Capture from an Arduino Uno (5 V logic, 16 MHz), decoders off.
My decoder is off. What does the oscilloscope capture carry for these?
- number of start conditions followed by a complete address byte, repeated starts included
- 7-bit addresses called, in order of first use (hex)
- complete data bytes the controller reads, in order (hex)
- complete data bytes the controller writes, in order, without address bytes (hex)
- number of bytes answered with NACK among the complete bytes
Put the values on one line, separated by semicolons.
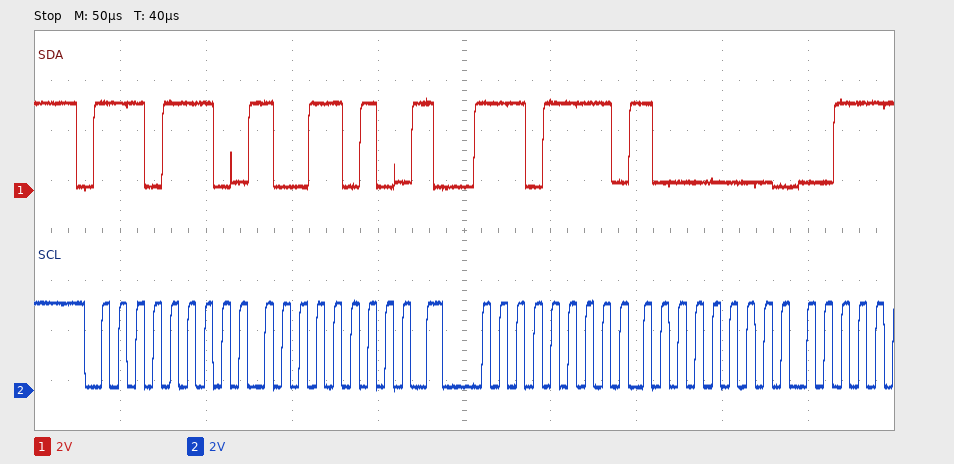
2; 0x77; 80; 9A; 0
